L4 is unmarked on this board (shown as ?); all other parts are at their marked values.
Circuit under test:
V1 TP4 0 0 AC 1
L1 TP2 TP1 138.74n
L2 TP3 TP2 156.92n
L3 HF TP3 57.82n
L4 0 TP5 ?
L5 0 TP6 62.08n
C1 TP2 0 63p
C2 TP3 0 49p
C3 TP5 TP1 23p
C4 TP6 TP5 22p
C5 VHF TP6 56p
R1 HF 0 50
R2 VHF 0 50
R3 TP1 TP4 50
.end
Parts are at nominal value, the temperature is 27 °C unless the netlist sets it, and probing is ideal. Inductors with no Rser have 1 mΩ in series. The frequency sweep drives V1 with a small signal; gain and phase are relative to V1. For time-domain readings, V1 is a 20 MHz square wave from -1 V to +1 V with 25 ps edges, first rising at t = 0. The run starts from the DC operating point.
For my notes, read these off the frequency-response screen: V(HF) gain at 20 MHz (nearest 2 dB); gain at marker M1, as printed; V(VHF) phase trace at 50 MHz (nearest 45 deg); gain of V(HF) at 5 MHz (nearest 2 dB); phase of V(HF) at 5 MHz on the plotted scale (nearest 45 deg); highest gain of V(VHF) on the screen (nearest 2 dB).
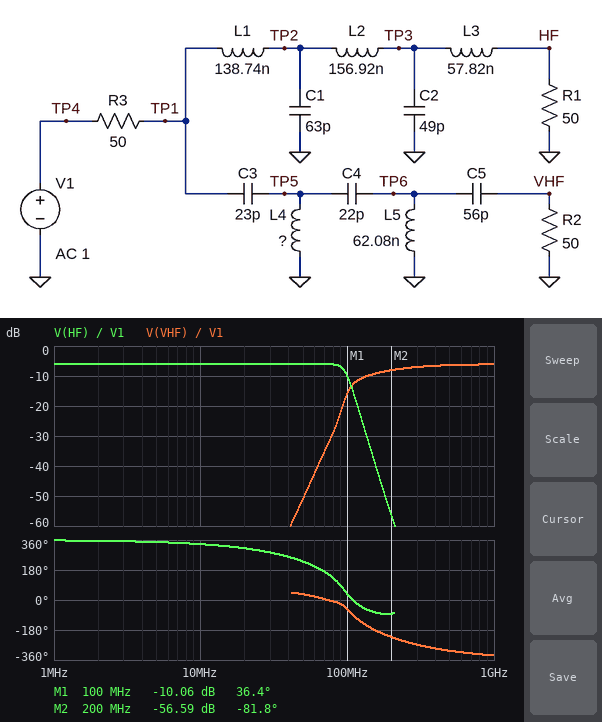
-6 dB
-10.06 dB
45 deg
-6 dB
360 deg
-6 dB
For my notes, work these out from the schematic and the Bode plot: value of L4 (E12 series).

18 nH
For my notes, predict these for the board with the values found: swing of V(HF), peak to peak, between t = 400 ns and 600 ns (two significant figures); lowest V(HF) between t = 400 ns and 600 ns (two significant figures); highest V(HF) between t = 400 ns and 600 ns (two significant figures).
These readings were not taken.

1.3 V
-670 mV
670 mV
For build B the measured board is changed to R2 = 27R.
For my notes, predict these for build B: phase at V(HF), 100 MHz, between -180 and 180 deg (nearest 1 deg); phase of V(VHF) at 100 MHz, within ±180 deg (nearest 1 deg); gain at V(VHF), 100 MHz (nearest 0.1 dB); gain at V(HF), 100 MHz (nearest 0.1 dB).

37 deg
-67 deg
-20.2 dB
-10.0 dB
